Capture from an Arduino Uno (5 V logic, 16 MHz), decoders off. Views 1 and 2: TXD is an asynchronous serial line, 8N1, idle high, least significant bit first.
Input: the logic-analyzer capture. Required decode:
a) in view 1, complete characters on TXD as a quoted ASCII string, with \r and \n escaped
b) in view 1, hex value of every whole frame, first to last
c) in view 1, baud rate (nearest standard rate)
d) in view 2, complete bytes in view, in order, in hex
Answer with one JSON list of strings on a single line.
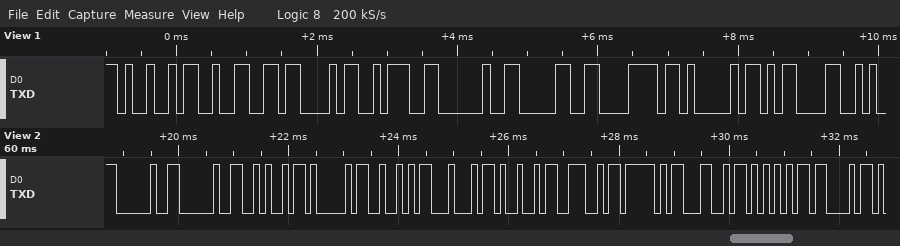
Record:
["\"I2C: 0xA\\r\"", "49 32 43 3A 20 30 78 41 0D", "9600 baud", "20 20 4A 41 52 44 49 4E 5F 4C 55 43"]
